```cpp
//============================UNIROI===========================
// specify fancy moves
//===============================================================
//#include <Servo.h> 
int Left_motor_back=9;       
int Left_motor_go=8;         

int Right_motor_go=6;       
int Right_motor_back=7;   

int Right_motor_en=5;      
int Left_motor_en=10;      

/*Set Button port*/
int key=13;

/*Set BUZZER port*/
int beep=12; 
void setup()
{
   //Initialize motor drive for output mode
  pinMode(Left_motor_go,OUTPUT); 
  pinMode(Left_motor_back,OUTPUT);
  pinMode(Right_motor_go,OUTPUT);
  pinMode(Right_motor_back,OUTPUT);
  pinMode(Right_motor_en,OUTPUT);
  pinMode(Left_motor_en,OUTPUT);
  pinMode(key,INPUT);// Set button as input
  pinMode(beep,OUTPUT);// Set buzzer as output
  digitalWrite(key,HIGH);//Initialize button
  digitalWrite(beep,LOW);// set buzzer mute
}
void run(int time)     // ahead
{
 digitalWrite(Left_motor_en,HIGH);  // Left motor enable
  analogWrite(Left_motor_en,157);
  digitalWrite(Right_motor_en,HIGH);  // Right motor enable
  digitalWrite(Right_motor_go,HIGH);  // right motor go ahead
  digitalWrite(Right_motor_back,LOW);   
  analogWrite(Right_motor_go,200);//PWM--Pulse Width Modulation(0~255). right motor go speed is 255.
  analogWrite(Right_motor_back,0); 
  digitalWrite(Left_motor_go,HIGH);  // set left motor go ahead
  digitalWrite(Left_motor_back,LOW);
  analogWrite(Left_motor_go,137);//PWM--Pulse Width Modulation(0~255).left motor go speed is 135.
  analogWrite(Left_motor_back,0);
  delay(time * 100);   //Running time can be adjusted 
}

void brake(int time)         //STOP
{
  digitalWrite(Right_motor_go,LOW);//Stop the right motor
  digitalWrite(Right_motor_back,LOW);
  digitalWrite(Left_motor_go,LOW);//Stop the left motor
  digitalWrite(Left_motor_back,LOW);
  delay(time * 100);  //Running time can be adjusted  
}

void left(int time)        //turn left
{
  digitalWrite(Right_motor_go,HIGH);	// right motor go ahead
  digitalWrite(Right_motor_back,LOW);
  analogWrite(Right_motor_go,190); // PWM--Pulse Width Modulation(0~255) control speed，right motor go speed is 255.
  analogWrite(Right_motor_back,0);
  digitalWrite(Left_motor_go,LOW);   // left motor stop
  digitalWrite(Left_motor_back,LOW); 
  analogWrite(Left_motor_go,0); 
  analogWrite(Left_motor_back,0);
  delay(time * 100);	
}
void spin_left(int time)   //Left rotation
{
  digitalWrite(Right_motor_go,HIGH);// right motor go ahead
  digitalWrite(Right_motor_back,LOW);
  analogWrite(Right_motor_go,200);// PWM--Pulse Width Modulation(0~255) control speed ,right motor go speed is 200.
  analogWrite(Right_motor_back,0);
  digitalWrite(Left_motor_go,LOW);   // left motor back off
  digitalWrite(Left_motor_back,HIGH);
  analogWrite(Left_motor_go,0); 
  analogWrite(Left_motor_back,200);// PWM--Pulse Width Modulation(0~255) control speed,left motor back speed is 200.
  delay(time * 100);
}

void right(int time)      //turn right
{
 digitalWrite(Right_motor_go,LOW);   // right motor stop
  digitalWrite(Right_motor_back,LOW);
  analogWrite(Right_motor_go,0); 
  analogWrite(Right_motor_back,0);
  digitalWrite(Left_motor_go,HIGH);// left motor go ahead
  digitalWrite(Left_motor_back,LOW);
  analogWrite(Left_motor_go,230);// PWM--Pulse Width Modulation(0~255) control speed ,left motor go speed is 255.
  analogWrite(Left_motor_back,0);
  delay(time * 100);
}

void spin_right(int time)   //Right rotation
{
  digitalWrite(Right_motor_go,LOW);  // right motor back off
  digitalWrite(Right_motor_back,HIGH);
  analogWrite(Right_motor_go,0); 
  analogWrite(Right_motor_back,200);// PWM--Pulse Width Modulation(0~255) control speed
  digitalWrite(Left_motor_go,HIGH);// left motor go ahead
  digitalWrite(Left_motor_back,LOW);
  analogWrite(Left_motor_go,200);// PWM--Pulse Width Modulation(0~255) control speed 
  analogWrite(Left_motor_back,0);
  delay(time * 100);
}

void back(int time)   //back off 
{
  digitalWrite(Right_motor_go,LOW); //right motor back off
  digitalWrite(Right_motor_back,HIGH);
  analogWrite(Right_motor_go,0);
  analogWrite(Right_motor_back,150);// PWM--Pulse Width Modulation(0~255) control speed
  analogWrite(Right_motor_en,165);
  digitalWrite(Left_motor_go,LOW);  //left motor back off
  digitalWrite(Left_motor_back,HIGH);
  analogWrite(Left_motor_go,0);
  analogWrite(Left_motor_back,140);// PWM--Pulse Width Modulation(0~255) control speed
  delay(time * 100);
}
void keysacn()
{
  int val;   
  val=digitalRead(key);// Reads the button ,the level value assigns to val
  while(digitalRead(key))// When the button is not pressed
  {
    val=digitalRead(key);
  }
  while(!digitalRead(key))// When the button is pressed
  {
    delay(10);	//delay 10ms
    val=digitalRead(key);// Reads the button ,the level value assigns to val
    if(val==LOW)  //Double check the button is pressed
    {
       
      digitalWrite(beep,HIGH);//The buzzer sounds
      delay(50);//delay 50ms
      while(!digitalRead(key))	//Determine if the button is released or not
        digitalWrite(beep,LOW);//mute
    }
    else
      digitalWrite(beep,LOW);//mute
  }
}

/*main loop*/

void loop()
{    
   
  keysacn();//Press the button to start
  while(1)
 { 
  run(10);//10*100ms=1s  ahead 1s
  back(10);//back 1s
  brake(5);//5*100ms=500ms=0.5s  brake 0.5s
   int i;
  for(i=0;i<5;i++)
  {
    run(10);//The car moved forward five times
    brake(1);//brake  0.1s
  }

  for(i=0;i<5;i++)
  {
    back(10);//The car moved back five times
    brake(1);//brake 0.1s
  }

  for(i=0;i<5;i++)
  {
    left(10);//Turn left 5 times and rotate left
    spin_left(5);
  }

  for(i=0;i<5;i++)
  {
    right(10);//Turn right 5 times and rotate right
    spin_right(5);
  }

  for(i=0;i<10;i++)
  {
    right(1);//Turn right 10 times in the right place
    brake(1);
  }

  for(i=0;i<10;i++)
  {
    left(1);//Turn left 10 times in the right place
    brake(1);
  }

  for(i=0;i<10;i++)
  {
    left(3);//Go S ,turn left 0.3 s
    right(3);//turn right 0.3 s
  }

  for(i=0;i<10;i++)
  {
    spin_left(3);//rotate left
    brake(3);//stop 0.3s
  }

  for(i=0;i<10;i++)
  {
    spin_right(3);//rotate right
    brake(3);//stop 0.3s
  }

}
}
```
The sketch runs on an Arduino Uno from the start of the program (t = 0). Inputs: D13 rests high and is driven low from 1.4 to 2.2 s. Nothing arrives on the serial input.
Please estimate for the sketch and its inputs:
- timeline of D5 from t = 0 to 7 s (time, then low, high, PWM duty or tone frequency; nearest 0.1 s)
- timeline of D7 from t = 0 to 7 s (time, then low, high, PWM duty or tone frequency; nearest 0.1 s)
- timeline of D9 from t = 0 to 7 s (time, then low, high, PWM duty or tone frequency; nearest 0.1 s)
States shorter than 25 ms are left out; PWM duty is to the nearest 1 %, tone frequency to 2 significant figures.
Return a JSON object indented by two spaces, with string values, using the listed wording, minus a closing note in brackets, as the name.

{
  "timeline of D5 from t = 0 to 7 s": "0 s low; 2.2 s high; 3.2 s PWM 65 %; 4.7 s high",
  "timeline of D7 from t = 0 to 7 s": "0 s low; 3.2 s high; 4.2 s low",
  "timeline of D9 from t = 0 to 7 s": "0 s low; 3.2 s PWM 55 %; 4.2 s low"
}
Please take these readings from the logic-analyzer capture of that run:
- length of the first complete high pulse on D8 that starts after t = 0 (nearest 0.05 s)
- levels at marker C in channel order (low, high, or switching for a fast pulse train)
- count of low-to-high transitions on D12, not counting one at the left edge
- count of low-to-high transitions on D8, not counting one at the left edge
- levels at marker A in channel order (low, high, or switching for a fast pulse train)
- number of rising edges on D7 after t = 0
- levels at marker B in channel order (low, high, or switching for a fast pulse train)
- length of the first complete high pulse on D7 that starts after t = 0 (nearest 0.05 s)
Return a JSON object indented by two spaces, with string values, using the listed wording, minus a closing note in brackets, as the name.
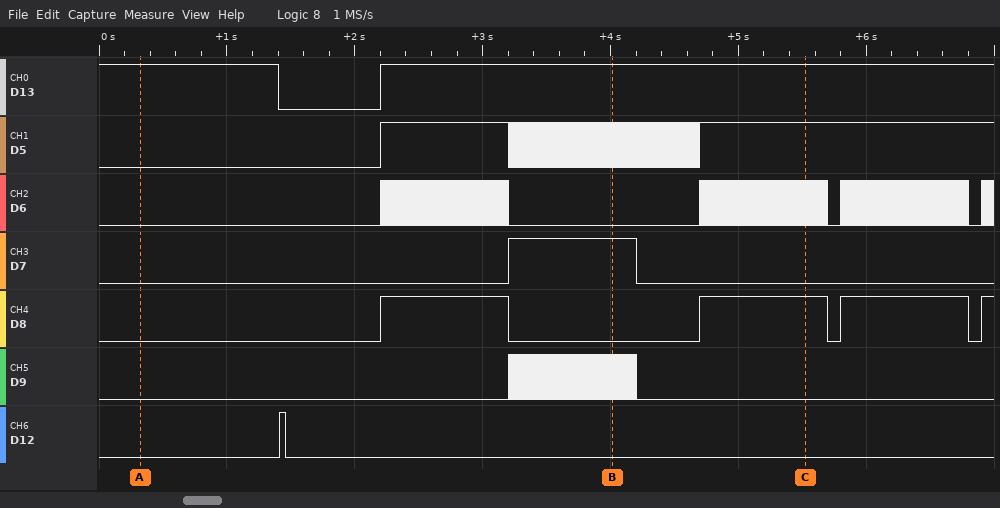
{
  "length of the first complete high pulse on D8 that starts after t = 0": "1.00 s",
  "levels at marker C in channel order": "D13 high, D5 high, D6 switching, D7 low, D8 high, D9 low, D12 low",
  "count of low-to-high transitions on D12, not counting one at the left edge": "1",
  "count of low-to-high transitions on D8, not counting one at the left edge": "4",
  "levels at marker A in channel order": "D13 high, D5 low, D6 low, D7 low, D8 low, D9 low, D12 low",
  "number of rising edges on D7 after t = 0": "1",
  "levels at marker B in channel order": "D13 high, D5 switching, D6 low, D7 high, D8 low, D9 switching, D12 low",
  "length of the first complete high pulse on D7 that starts after t = 0": "1.00 s"
}
